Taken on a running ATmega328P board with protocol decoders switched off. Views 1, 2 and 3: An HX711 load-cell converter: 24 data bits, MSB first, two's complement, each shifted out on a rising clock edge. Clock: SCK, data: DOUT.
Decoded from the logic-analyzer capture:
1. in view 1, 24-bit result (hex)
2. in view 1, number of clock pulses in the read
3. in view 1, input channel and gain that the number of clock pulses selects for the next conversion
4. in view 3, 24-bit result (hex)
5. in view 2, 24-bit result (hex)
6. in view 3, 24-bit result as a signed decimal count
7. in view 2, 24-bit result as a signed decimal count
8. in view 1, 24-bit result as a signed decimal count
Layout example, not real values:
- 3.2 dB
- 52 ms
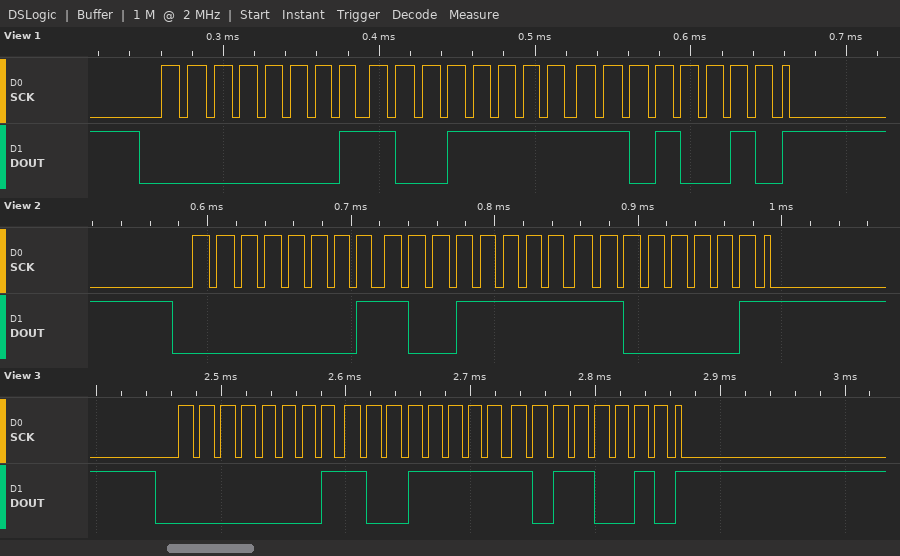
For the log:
- 0x019FD2
- 25
- channel A, gain 128
- 0x019FB2
- 0x019FC1
- 106418
- 106433
- 106450
